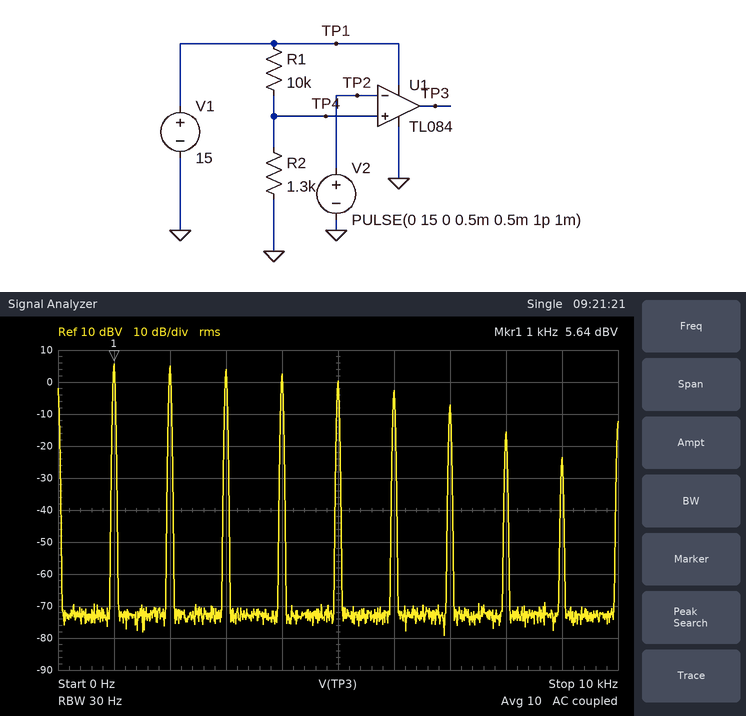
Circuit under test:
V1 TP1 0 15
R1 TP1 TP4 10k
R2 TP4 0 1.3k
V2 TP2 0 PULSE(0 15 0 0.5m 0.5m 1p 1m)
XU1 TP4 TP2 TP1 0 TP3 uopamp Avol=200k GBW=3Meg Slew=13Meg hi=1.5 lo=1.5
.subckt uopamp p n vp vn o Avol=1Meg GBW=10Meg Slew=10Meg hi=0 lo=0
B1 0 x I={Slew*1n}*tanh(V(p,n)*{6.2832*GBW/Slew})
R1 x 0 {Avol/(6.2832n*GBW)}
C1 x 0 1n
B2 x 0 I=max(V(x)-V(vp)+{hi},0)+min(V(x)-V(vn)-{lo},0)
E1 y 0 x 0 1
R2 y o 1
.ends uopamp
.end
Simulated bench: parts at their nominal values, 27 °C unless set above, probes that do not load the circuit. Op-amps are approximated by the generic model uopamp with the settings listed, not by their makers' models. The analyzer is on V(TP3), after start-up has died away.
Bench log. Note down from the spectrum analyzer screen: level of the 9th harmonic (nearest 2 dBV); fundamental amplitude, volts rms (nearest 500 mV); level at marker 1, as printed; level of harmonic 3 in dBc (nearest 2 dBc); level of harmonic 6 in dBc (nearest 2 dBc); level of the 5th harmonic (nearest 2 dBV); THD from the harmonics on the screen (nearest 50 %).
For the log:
-24 dBV
2.0 V
5.64 dBV
-2 dBc
-8 dBc
0 dBV
150 %
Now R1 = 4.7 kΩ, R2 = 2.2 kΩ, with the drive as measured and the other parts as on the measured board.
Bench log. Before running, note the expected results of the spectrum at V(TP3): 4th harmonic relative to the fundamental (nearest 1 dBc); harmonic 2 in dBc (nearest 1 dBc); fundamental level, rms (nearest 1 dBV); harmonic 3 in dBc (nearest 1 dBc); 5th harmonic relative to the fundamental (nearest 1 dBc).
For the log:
-13 dBc
-5 dBc
13 dBV
-25 dBc
-13 dBc
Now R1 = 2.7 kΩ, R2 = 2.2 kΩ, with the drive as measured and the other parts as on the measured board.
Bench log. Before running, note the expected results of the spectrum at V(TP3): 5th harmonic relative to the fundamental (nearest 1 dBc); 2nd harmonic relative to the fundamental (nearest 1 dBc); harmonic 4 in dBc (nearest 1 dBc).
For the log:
-17 dBc
-16 dBc
-16 dBc
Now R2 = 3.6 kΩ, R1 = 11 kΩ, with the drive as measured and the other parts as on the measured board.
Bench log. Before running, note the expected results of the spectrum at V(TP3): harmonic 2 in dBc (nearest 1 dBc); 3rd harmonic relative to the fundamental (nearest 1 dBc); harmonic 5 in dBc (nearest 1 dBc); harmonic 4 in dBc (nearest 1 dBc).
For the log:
-3 dBc
-9 dBc
-14 dBc
-36 dBc
